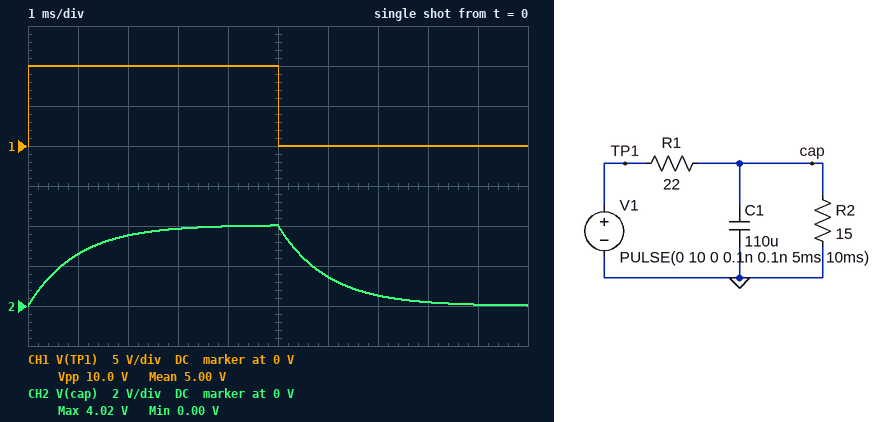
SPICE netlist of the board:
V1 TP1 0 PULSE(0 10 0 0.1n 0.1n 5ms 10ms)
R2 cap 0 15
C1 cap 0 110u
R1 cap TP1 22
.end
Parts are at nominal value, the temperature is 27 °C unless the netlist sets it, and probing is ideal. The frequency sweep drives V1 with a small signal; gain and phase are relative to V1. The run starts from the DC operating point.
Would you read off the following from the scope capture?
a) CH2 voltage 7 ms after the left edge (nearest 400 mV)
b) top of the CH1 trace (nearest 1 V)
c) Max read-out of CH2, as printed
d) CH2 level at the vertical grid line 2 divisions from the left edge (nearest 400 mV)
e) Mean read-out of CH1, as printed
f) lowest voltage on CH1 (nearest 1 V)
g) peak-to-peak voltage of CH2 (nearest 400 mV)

400 mV
10 V
4.02 V
3.6 V
5.00 V
0 V
4.0 V
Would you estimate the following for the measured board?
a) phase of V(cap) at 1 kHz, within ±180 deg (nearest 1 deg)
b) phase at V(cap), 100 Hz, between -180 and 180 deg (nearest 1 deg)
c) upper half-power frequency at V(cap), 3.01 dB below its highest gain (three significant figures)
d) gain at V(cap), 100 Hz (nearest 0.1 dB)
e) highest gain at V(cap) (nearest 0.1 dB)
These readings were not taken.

-81 deg
-32 deg
162 Hz
-9.2 dB
-7.8 dB
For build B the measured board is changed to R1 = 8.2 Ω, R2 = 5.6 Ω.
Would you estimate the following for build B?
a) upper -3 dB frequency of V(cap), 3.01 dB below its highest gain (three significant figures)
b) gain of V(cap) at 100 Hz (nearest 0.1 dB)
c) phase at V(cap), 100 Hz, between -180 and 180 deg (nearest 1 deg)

435 Hz
-8.1 dB
-13 deg
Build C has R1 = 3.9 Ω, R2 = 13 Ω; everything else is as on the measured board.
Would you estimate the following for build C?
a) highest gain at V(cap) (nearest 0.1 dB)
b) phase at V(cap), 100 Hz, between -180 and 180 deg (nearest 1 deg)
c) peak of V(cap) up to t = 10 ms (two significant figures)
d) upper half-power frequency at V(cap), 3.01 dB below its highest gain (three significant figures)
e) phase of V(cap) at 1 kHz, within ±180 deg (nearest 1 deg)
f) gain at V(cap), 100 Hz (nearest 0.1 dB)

-2.3 dB
-12 deg
7.7 V
482 Hz
-64 deg
-2.5 dB
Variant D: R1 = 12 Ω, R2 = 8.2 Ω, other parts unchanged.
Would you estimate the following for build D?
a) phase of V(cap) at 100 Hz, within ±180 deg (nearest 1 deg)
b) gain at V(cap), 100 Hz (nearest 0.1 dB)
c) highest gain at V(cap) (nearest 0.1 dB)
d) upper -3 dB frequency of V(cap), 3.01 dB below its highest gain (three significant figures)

-19 deg
-8.3 dB
-7.8 dB
297 Hz
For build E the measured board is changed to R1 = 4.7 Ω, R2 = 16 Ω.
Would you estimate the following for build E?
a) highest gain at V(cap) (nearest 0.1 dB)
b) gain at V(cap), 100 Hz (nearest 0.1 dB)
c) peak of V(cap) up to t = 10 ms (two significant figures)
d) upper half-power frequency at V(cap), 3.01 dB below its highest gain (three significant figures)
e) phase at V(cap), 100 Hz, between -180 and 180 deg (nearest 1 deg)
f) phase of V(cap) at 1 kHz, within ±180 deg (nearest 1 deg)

-2.2 dB
-2.5 dB
7.7 V
398 Hz
-14 deg
-68 deg
